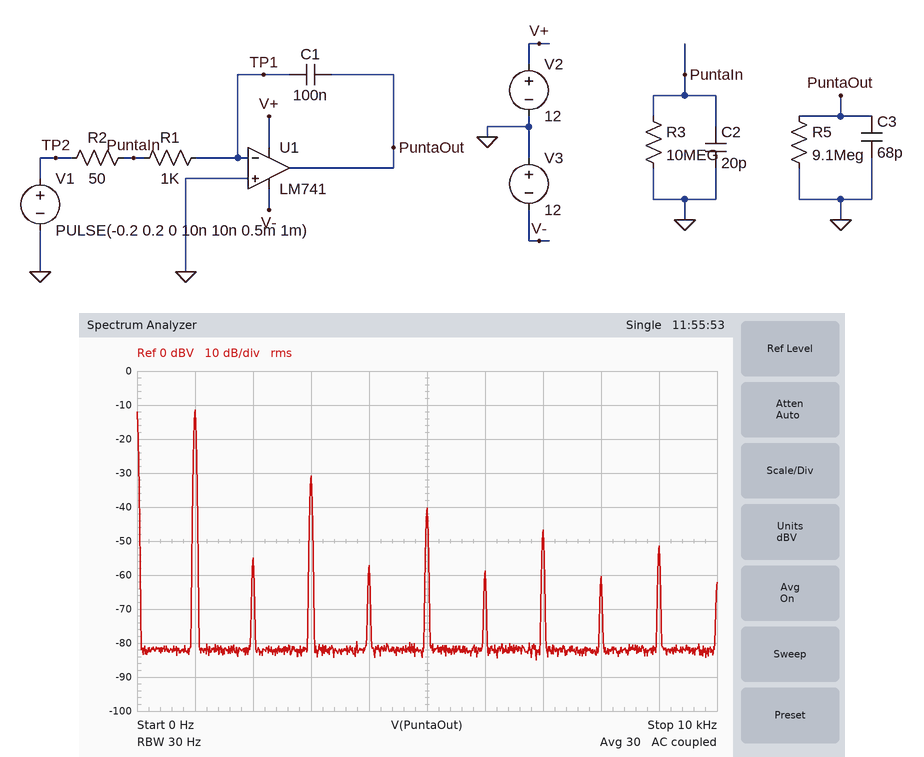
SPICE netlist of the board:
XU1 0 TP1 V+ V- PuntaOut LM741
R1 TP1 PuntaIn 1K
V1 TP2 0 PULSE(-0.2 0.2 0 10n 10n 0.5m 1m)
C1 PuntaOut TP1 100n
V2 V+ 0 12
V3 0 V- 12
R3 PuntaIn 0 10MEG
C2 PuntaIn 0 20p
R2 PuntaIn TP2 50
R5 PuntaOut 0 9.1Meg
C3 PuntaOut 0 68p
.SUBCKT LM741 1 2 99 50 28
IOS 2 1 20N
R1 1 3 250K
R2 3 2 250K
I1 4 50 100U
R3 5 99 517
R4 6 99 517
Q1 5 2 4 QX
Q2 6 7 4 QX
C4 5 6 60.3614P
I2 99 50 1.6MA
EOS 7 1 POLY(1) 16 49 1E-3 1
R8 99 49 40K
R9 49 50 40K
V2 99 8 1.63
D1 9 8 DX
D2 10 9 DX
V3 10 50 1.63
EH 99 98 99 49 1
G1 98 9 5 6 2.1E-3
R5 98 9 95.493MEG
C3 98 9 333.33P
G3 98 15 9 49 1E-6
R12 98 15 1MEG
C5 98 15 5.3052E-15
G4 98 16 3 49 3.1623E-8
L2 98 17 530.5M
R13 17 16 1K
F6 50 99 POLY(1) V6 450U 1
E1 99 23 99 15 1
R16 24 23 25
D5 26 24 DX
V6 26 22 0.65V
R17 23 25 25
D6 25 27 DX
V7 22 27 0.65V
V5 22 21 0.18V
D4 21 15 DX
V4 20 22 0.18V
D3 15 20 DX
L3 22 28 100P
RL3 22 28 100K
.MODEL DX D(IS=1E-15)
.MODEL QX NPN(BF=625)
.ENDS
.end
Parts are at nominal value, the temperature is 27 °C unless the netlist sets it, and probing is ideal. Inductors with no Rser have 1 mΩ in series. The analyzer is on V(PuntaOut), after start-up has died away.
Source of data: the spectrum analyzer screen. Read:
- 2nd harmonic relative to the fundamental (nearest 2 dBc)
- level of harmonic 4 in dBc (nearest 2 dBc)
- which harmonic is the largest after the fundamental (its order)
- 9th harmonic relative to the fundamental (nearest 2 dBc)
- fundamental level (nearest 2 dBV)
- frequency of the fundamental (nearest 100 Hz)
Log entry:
-44 dBc
-46 dBc
3
-40 dBc
-12 dBV
1.0 kHz
